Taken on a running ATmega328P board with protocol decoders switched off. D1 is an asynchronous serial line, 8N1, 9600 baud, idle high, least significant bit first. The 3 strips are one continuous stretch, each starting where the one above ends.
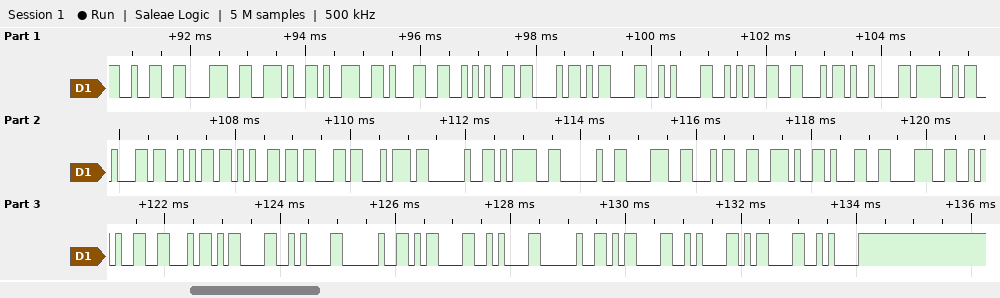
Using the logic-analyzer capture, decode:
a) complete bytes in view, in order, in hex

32 38 2E 39 31 2A 43 0D 0A 2A 46 09 4F 62 6A 65 63 74 20 3D 20 38 34 2E 31 38 2A 46 0D 0A 20 0D 0A 20 0D 0A 0D 0A
